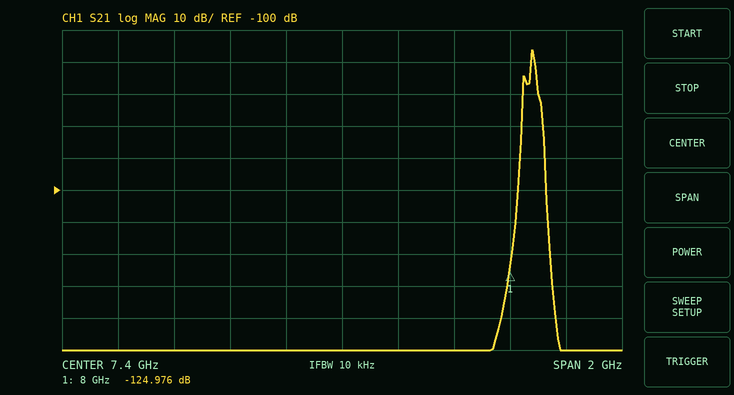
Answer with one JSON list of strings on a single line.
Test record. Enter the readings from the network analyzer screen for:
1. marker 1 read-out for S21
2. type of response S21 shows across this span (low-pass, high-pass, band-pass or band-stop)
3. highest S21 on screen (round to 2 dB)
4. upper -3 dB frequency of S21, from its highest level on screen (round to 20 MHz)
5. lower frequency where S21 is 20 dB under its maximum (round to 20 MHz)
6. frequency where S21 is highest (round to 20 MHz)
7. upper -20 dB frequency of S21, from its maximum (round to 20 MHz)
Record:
["-124.976 dB", "band-pass", "-56 dB", "8.08 GHz", "8.04 GHz", "8.08 GHz", "8.12 GHz"]
